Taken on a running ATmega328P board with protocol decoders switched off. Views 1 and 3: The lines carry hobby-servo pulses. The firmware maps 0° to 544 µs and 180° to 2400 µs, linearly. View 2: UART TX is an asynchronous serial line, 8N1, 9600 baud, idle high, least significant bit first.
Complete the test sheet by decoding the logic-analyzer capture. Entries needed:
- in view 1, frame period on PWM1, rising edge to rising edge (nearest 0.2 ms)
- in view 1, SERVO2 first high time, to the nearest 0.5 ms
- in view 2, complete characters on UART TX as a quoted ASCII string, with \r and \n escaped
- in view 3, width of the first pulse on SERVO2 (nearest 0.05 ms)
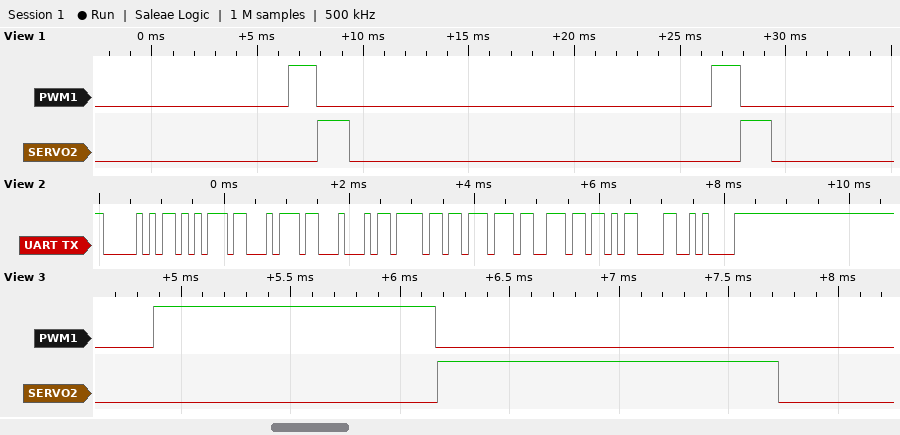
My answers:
20.0 ms
1.5 ms
"PutDown\r\n"
1.55 ms
